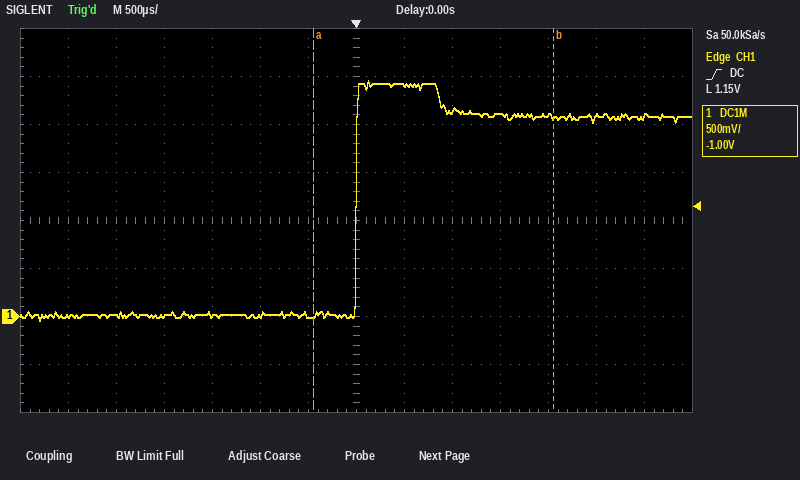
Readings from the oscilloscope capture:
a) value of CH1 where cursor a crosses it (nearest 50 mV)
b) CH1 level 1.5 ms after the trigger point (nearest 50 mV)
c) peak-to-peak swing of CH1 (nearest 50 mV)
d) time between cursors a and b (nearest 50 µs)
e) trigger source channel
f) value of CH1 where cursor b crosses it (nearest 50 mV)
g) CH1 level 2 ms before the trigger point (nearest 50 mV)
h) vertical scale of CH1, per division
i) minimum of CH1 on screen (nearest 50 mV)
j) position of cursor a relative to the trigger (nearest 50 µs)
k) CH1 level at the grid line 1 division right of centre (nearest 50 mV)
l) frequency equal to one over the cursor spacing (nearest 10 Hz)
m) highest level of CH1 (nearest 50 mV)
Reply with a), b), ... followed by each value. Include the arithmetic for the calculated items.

a) 0 mV
b) 2.10 V
c) 2.45 V − (-50 mV) = 2.50 V
d) 2.50 ms
e) CH1
f) 2.10 V
g) 0 mV
h) 500 mV
i) -50 mV
j) -450 µs
k) 2.40 V
l) 1 / 2.50 ms ≈ 400 Hz
m) 2.45 V
